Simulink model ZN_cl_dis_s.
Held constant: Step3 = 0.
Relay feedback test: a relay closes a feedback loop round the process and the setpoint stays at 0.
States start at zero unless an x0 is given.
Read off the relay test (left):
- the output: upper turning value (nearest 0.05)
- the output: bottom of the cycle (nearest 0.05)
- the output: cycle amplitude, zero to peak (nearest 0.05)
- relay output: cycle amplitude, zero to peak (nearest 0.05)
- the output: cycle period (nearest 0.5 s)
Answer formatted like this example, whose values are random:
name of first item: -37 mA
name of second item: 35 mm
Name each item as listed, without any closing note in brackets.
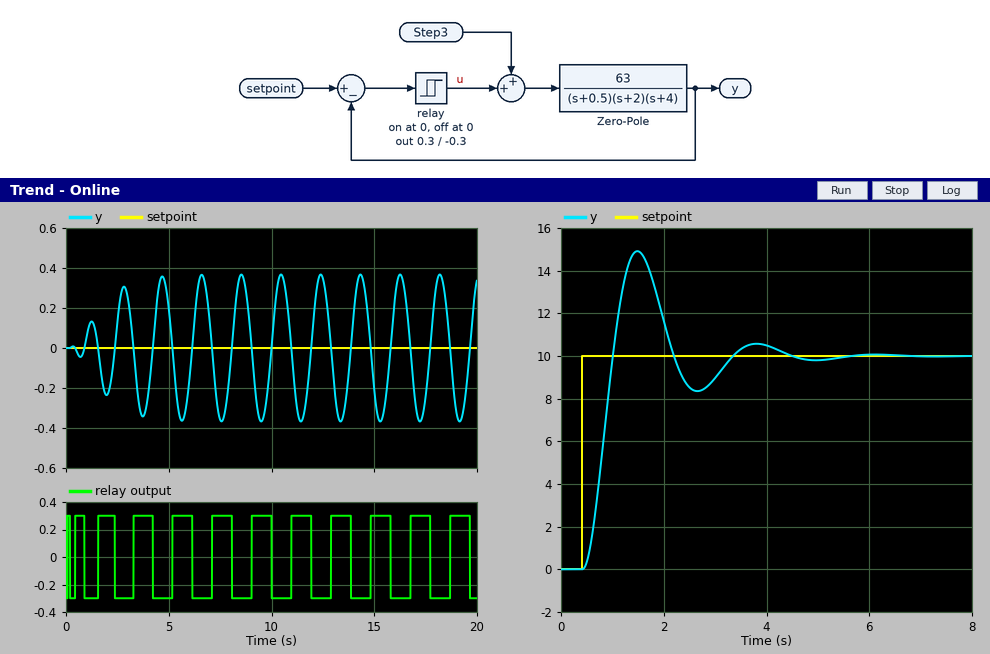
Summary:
the output: upper turning value: 0.35
the output: bottom of the cycle: -0.35
the output: cycle amplitude, zero to peak: 0.35
relay output: cycle amplitude, zero to peak: 0.30
the output: cycle period: 2.0 s
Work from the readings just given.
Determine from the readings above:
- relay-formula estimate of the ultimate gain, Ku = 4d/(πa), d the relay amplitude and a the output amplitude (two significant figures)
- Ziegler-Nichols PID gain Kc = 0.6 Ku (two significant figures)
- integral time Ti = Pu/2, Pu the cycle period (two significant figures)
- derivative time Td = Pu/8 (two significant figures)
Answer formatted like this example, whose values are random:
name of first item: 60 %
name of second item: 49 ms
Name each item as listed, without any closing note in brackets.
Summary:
relay-formula estimate of the ultimate gain, Ku = 4d/(πa), d the relay amplitude and a the output amplitude: 1.1
Ziegler-Nichols PID gain Kc = 0.6 Ku: 0.66
integral time Ti = Pu/2, Pu the cycle period: 1.0 s
derivative time Td = Pu/8: 0.25 s
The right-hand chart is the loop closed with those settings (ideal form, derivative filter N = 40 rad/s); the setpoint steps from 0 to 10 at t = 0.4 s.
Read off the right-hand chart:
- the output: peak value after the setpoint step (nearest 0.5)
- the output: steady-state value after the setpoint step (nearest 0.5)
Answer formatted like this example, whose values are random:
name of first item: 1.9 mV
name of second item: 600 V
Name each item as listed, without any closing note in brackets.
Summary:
the output: peak value after the setpoint step: 15.0
the output: steady-state value after the setpoint step: 10.0
